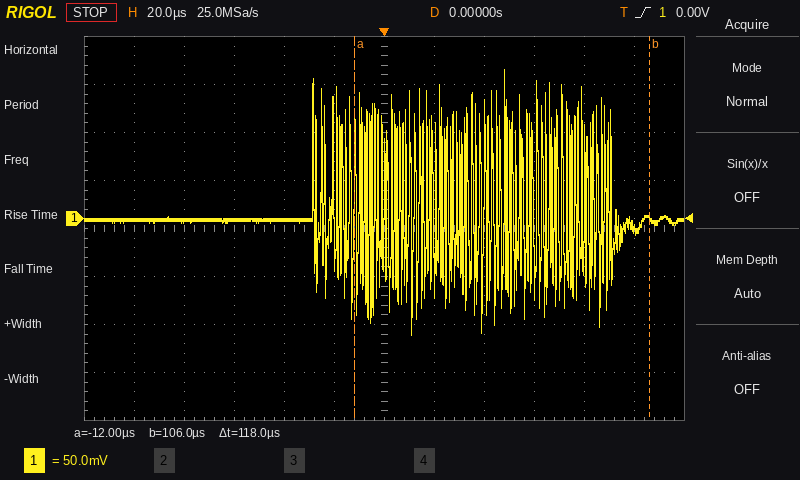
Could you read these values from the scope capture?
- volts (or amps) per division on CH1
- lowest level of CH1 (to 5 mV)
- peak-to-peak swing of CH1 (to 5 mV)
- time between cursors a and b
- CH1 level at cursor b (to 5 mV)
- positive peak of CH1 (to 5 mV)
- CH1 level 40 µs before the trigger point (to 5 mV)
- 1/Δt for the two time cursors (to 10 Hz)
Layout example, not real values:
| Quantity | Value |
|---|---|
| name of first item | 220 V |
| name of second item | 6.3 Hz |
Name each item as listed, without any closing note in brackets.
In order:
| Quantity | Value |
|---|---|
| volts (or amps) per division on CH1 | 50 mV |
| lowest level of CH1 | -120 mV |
| peak-to-peak swing of CH1 | 275 mV |
| time between cursors a and b | 118 µs |
| CH1 level at cursor b | 0 mV |
| positive peak of CH1 | 155 mV |
| CH1 level 40 µs before the trigger point | 0 mV |
| 1/Δt for the two time cursors | 8.47 kHz |
